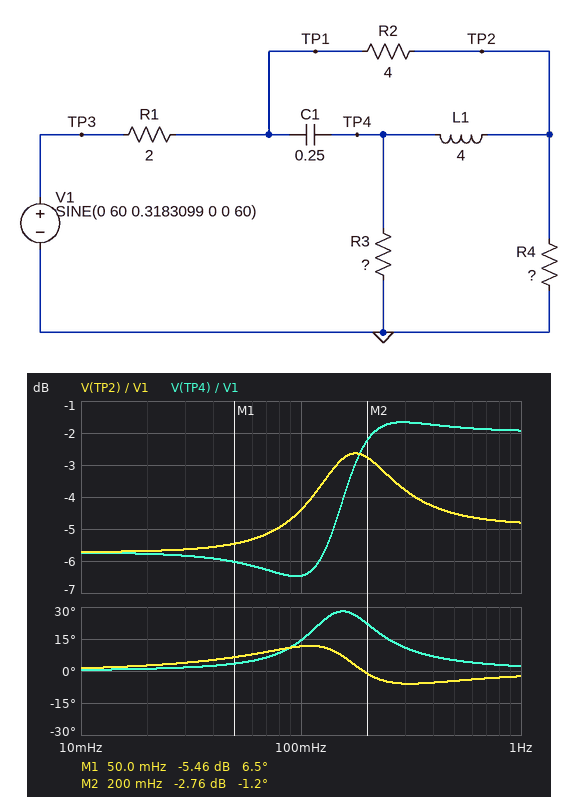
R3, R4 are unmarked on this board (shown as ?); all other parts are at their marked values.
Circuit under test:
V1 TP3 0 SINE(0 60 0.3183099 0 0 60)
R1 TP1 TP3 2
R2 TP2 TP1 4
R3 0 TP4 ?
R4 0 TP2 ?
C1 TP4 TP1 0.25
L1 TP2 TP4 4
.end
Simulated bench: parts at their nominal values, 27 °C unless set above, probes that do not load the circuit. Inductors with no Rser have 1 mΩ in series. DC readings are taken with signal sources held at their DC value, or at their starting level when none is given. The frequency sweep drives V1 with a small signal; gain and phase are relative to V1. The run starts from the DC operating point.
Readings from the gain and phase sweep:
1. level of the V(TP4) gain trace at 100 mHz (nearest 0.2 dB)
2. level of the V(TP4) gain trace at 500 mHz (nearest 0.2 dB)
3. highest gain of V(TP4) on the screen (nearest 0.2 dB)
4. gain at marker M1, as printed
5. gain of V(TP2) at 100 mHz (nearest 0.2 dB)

-6.4 dB
-1.8 dB
-1.6 dB
-5.46 dB
-4.4 dB
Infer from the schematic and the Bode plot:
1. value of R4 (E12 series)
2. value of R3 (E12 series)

10 Ω
18 Ω
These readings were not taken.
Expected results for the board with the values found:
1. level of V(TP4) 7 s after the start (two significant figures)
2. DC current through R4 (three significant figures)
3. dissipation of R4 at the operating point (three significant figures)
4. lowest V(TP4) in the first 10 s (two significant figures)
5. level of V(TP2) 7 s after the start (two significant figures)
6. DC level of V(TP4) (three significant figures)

23 V
2.69 A
72.2 W
-50 V
26 V
26.9 V
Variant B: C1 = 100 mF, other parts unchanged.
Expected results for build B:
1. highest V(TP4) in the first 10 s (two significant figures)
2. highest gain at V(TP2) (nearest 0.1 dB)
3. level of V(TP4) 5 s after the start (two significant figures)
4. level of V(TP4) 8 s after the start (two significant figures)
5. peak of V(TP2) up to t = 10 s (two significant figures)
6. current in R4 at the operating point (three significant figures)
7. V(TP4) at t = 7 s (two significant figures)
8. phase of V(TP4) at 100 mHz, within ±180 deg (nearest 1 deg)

45 V
-2.9 dB
-37 V
-43 V
43 V
2.69 A
5.4 V
-1 deg
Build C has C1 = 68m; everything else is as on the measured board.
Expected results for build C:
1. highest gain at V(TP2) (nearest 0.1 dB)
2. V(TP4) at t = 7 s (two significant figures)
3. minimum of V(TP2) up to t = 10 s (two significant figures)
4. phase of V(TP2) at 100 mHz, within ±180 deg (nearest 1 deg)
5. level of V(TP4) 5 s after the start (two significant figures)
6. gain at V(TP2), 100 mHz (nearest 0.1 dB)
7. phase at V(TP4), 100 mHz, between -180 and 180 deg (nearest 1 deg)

-3.1 dB
-3.8 V
-42 V
5 deg
-21 V
-5.6 dB
-3 deg
